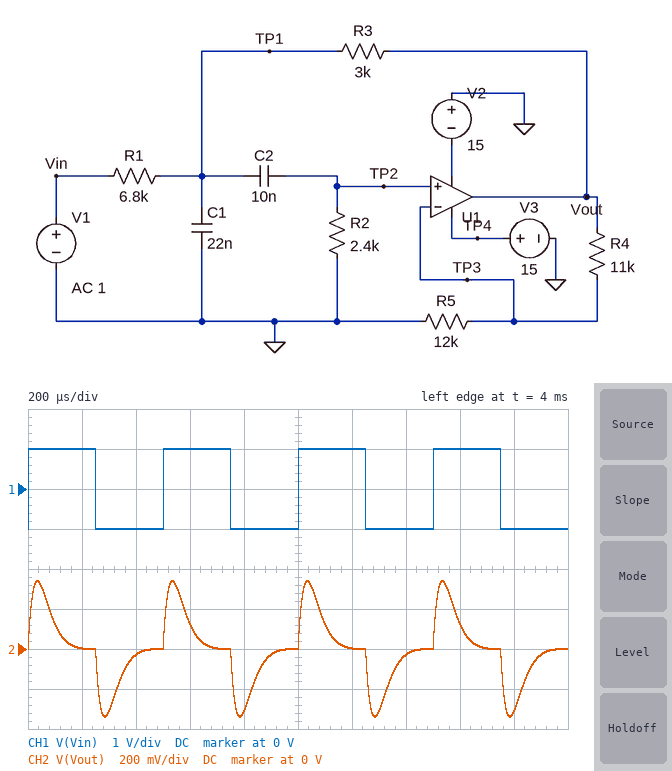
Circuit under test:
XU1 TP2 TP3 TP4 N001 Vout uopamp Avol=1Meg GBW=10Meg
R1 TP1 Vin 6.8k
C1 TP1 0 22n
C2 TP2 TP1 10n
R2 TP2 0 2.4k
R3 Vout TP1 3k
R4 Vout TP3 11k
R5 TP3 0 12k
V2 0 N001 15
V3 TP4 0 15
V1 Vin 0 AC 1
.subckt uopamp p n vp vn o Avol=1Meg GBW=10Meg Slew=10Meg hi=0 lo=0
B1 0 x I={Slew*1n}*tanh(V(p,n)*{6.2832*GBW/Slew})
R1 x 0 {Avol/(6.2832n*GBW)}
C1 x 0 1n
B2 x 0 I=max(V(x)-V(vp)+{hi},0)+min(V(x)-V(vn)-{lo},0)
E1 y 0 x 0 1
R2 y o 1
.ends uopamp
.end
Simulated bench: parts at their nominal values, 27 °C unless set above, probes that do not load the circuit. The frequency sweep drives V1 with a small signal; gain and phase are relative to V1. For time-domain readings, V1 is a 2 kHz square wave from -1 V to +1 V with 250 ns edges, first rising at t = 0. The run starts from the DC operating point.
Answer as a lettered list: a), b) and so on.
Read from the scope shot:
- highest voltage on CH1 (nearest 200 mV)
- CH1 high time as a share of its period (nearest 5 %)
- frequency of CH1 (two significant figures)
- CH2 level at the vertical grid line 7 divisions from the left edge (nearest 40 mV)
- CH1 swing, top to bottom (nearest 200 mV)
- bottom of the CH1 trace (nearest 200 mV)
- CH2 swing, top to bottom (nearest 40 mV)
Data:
a) 1.0 V
b) 50 %
c) 2.0 kHz
d) -40 mV
e) 2.0 V
f) -1.0 V
g) 680 mV
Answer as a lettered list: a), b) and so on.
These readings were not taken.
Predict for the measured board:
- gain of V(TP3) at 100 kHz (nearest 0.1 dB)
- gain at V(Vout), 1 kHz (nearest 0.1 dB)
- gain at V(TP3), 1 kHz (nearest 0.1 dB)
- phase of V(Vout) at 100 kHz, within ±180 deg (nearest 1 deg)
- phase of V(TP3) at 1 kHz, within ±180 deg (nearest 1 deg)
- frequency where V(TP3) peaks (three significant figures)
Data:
a) -39.5 dB
b) -21.3 dB
c) -26.9 dB
d) -86 deg
e) 69 deg
f) 4.80 kHz
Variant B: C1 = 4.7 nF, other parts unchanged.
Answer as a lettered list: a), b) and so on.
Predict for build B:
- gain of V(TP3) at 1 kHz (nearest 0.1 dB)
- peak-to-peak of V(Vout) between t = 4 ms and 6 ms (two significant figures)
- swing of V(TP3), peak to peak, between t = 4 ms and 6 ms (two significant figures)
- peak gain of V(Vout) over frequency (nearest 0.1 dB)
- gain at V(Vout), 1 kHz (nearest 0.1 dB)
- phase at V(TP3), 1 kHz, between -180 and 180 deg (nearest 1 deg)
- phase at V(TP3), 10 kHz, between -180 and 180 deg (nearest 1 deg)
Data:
a) -26.7 dB
b) 1.6 V
c) 850 mV
d) -4.1 dB
e) -21.1 dB
f) 82 deg
g) 3 deg
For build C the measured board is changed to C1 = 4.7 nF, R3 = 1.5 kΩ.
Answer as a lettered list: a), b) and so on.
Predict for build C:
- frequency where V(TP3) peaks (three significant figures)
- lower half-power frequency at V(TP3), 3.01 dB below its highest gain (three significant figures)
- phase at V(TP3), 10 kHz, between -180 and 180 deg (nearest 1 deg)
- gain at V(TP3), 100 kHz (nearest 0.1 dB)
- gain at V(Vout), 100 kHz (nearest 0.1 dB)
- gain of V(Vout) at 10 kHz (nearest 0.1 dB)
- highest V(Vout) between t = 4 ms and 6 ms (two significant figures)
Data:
a) 13.5 kHz
b) 11.2 kHz
c) 58 deg
d) -26.0 dB
e) -20.3 dB
f) -0.1 dB
g) 1.1 V
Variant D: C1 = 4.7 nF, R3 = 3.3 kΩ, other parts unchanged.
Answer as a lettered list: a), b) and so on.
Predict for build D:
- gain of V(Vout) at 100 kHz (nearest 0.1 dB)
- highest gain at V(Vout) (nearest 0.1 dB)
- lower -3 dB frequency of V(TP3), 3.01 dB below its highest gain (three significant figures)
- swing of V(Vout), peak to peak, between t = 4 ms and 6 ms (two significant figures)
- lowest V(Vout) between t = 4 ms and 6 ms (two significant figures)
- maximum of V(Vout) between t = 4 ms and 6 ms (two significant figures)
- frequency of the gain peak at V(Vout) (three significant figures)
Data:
a) -20.5 dB
b) -4.7 dB
c) 4.79 kHz
d) 1.6 V
e) -800 mV
f) 800 mV
g) 10.0 kHz
